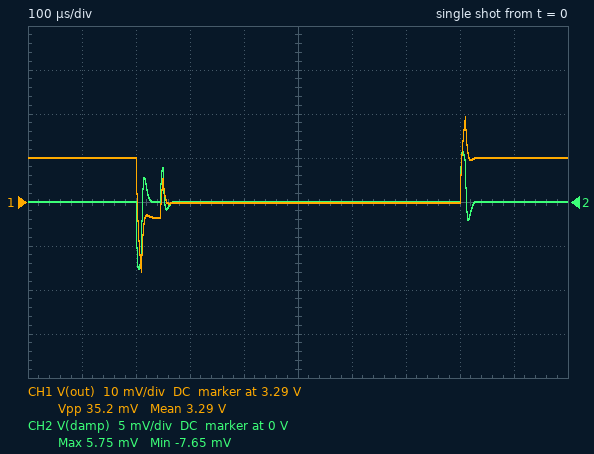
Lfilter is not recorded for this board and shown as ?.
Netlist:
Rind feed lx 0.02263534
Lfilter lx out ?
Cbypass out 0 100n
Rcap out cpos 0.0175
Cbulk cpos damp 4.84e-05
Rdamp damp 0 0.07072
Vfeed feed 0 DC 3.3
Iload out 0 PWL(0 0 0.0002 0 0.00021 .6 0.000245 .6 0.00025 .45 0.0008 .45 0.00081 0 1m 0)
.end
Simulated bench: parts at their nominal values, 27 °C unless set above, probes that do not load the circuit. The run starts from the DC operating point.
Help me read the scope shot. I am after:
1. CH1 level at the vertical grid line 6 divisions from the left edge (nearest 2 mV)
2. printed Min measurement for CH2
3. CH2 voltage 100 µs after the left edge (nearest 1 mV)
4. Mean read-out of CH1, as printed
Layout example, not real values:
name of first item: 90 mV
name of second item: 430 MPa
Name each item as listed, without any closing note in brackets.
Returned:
CH1 level at the vertical grid line 6 divisions from the left edge: 3.290 V
printed Min measurement for CH2: -7.65 mV
CH2 voltage 100 µs after the left edge: 0 V
Mean read-out of CH1, as printed: 3.29 V
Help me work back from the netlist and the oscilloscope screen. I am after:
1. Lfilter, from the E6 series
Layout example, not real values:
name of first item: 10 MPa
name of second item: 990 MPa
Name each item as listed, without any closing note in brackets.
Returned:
Lfilter, from the E6 series: 220 nH
